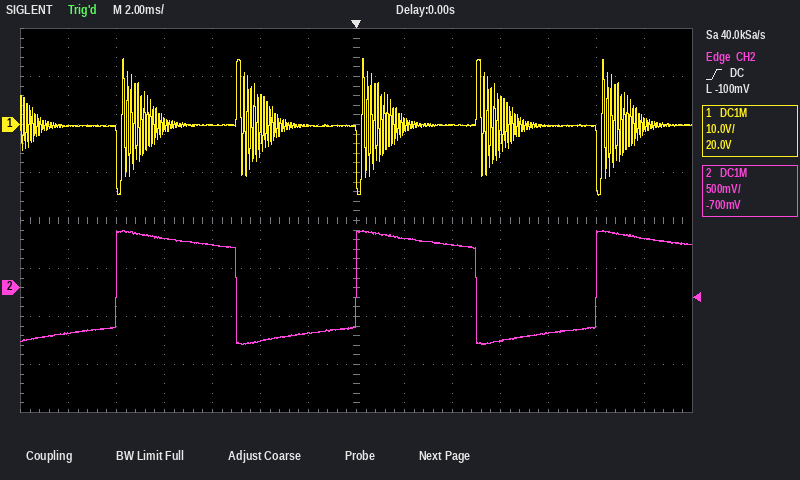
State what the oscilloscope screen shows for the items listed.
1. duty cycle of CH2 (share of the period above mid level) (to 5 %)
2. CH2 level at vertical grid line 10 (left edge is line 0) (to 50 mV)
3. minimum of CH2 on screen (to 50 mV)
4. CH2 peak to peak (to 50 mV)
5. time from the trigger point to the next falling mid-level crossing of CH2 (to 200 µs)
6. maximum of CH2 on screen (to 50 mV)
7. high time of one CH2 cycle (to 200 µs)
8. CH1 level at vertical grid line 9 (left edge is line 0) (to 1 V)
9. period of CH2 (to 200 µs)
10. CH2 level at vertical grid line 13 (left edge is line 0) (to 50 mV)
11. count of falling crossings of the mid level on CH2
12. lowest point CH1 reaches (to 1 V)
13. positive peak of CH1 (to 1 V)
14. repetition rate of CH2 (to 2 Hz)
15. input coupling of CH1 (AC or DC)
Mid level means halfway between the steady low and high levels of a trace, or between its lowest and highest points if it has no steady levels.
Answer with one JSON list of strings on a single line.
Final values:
["50 %", "-550 mV", "-600 mV", "1.20 V", "5.0 ms", "600 mV", "5.0 ms", "0 V", "10.0 ms", "500 mV", "2", "-15 V", "14 V", "100 Hz", "DC"]
